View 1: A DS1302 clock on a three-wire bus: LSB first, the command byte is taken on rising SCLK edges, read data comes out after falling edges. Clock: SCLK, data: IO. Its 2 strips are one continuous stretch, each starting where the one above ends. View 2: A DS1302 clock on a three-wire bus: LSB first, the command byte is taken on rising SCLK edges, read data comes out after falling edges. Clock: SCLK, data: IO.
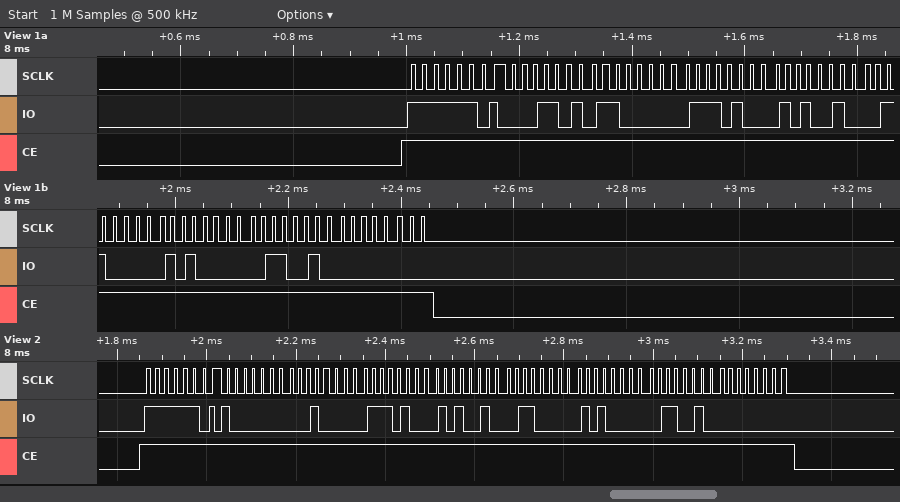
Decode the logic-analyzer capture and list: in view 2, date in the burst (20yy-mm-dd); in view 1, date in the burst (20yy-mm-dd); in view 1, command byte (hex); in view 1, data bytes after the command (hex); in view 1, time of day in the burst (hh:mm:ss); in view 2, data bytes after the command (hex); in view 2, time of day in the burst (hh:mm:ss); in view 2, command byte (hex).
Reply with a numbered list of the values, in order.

1. 2026-06-25
2. 2026-06-25
3. 0xBF
4. 58 03 17 25 06 05 26 00
5. 17:03:58
6. 01 04 17 25 06 05 26 00
7. 17:04:01
8. 0xBF
